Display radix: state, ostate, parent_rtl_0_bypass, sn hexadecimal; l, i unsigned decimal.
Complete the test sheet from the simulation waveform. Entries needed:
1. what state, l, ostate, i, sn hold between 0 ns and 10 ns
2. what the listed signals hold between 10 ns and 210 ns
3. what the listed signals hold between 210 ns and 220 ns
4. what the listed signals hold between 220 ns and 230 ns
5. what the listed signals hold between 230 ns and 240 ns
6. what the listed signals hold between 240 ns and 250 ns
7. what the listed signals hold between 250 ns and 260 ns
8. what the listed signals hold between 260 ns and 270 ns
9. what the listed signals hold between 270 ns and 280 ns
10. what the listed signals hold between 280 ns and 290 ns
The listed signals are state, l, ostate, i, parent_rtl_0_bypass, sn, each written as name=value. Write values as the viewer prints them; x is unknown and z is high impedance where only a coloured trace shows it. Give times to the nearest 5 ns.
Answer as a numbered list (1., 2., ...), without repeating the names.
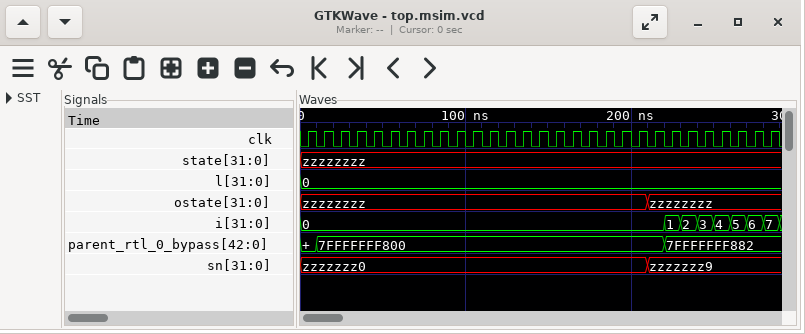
1. state=zzzzzzzz, l=0, ostate=zzzzzzzz, i=0, sn=zzzzzzz0
2. state=zzzzzzzz, l=0, ostate=zzzzzzzz, i=0, parent_rtl_0_bypass=7FFFFFFF800, sn=zzzzzzz0
3. state=zzzzzzzz, l=0, ostate=zzzzzzzz, i=0, parent_rtl_0_bypass=7FFFFFFF800, sn=zzzzzzz9
4. state=zzzzzzzz, l=0, ostate=zzzzzzzz, i=1, parent_rtl_0_bypass=7FFFFFFF882, sn=zzzzzzz9
5. state=zzzzzzzz, l=0, ostate=zzzzzzzz, i=2, parent_rtl_0_bypass=7FFFFFFF882, sn=zzzzzzz9
6. state=zzzzzzzz, l=0, ostate=zzzzzzzz, i=3, parent_rtl_0_bypass=7FFFFFFF882, sn=zzzzzzz9
7. state=zzzzzzzz, l=0, ostate=zzzzzzzz, i=4, parent_rtl_0_bypass=7FFFFFFF882, sn=zzzzzzz9
8. state=zzzzzzzz, l=0, ostate=zzzzzzzz, i=5, parent_rtl_0_bypass=7FFFFFFF882, sn=zzzzzzz9
9. state=zzzzzzzz, l=0, ostate=zzzzzzzz, i=6, parent_rtl_0_bypass=7FFFFFFF882, sn=zzzzzzz9
10. state=zzzzzzzz, l=0, ostate=zzzzzzzz, i=7, parent_rtl_0_bypass=7FFFFFFF882, sn=zzzzzzz9
